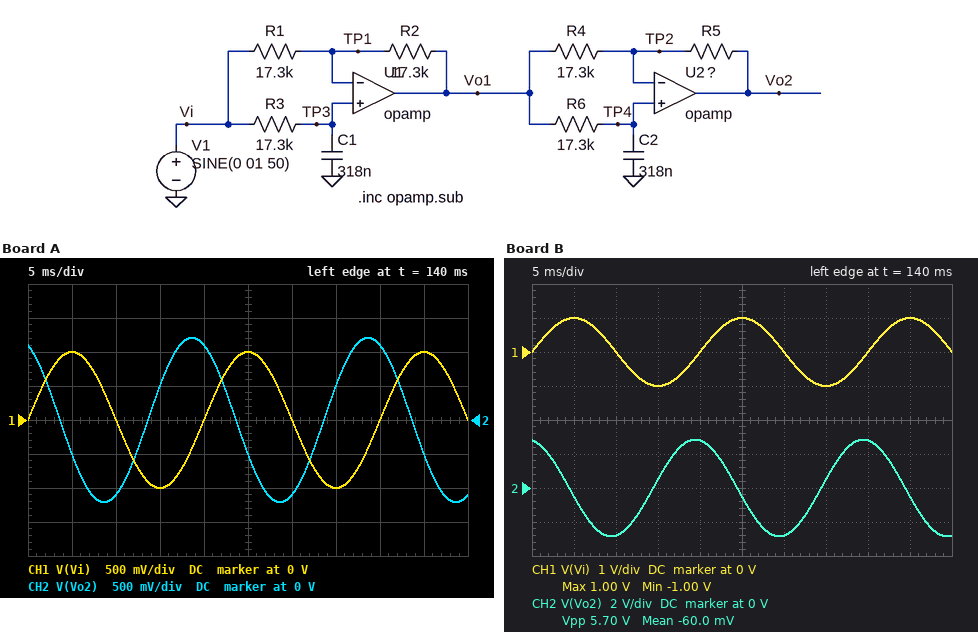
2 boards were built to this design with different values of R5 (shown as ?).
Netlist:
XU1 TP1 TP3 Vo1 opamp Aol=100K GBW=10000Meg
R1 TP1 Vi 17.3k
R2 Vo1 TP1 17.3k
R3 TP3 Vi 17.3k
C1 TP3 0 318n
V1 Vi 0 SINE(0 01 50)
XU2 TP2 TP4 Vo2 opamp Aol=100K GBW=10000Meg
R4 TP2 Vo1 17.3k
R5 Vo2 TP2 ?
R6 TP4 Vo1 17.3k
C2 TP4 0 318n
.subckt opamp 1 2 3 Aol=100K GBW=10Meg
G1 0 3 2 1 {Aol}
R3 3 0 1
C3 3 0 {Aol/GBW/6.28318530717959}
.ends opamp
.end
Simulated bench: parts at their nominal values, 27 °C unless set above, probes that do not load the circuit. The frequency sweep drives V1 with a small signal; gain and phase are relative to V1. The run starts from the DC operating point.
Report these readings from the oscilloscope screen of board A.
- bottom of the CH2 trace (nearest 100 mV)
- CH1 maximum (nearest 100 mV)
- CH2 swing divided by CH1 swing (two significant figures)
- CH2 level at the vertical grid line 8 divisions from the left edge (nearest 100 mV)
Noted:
-1.2 V
1.0 V
1.2
1.1 V
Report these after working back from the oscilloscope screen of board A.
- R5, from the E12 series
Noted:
22 kΩ
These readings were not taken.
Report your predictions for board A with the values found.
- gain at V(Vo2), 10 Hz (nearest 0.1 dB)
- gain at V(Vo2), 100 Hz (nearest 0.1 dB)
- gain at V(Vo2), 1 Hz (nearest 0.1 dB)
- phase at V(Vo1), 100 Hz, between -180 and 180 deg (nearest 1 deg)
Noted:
0.3 dB
2.0 dB
0 dB
-148 deg
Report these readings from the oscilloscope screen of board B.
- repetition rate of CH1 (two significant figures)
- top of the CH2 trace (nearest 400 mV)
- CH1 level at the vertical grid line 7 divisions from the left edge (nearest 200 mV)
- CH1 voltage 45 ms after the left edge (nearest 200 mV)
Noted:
50 Hz
2.8 V
-1.0 V
1.0 V
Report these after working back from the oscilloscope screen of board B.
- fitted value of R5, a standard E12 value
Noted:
56 kΩ
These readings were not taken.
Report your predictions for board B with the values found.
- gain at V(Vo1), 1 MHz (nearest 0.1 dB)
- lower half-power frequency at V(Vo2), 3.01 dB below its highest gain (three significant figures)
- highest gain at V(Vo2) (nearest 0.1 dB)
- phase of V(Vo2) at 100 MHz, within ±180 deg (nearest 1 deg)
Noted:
0 dB
26.0 Hz
10.2 dB
-4 deg
